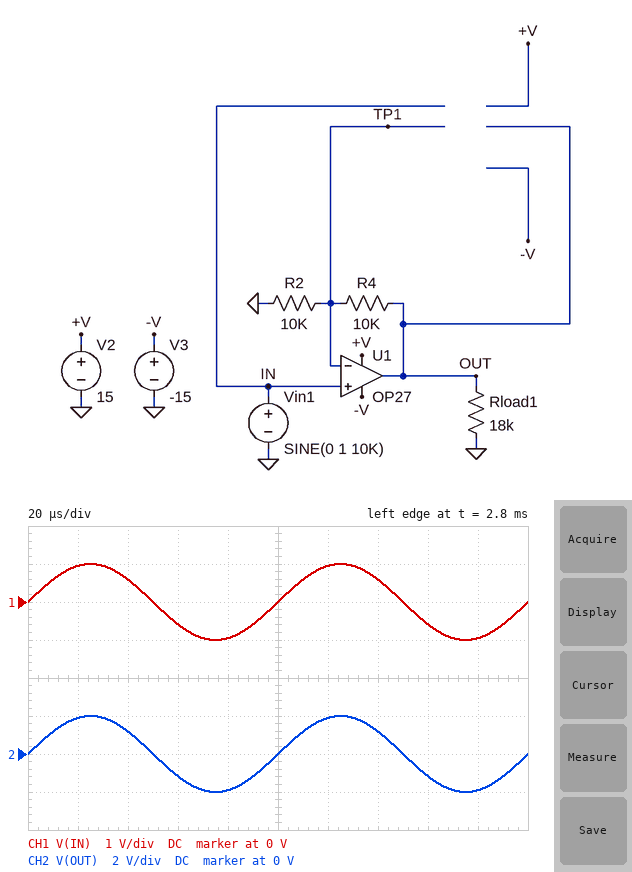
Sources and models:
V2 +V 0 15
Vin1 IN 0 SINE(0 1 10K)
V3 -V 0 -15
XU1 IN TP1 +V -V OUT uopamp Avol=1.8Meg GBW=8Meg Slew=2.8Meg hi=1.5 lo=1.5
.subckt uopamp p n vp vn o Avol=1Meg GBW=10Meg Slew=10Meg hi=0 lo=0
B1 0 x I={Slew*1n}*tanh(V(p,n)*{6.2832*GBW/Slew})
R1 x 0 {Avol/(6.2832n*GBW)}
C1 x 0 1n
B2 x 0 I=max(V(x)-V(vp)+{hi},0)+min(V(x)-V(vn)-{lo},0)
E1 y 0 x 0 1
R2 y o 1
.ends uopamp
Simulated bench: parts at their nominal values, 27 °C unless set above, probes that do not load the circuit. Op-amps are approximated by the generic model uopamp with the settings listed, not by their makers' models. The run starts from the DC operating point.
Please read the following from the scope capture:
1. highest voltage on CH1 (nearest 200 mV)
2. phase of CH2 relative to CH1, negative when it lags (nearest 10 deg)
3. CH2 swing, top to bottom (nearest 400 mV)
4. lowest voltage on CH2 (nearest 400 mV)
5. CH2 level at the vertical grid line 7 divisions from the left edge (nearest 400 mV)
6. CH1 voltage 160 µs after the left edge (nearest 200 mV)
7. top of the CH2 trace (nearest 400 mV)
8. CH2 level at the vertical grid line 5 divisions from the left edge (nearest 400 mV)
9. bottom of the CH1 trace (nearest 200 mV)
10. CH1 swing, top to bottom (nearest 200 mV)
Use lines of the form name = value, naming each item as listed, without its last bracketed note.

highest voltage on CH1 = 1.0 V
phase of CH2 relative to CH1, negative when it lags = 0 deg
CH2 swing, top to bottom = 4.0 V
lowest voltage on CH2 = -2.0 V
CH2 level at the vertical grid line 7 divisions from the left edge = 1.2 V
CH1 voltage 160 µs after the left edge = -600 mV
top of the CH2 trace = 2.0 V
CH2 level at the vertical grid line 5 divisions from the left edge = 0 V
bottom of the CH1 trace = -1.0 V
CH1 swing, top to bottom = 2.0 V
